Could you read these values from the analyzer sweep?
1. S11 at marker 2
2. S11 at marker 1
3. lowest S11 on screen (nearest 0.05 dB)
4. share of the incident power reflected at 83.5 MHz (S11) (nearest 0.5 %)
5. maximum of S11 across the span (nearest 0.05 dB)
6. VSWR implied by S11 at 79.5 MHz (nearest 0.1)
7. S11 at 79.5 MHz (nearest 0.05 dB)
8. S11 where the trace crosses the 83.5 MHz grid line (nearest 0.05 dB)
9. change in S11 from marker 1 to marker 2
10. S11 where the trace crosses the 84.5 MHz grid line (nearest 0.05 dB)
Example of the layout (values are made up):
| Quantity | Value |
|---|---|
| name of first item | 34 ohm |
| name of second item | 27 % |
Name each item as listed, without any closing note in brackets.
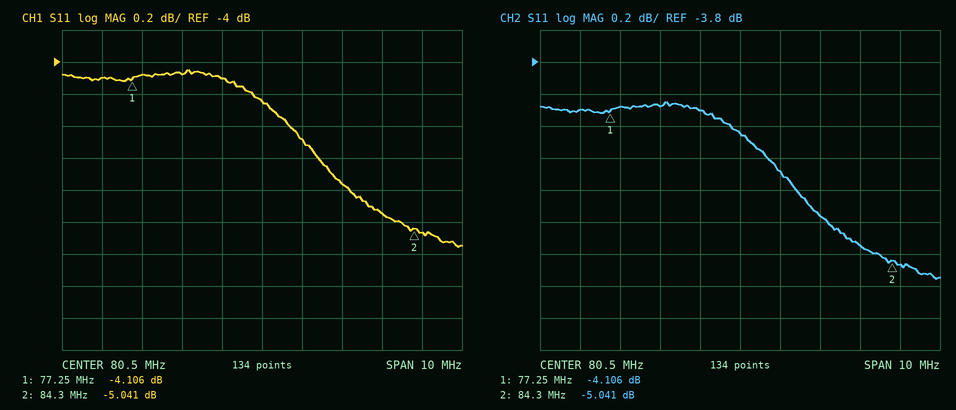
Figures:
| Quantity | Value |
|---|---|
| S11 at marker 2 | -5.041 dB |
| S11 at marker 1 | -4.106 dB |
| lowest S11 on screen | -5.15 dB |
| share of the incident power reflected at 83.5 MHz (S11) | 32.0 % |
| maximum of S11 across the span | -4.05 dB |
| VSWR implied by S11 at 79.5 MHz | 4.3 |
| S11 at 79.5 MHz | -4.10 dB |
| S11 where the trace crosses the 83.5 MHz grid line | -4.95 dB |
| change in S11 from marker 1 to marker 2 | -0.935 dB |
| S11 where the trace crosses the 84.5 MHz grid line | -5.05 dB |
